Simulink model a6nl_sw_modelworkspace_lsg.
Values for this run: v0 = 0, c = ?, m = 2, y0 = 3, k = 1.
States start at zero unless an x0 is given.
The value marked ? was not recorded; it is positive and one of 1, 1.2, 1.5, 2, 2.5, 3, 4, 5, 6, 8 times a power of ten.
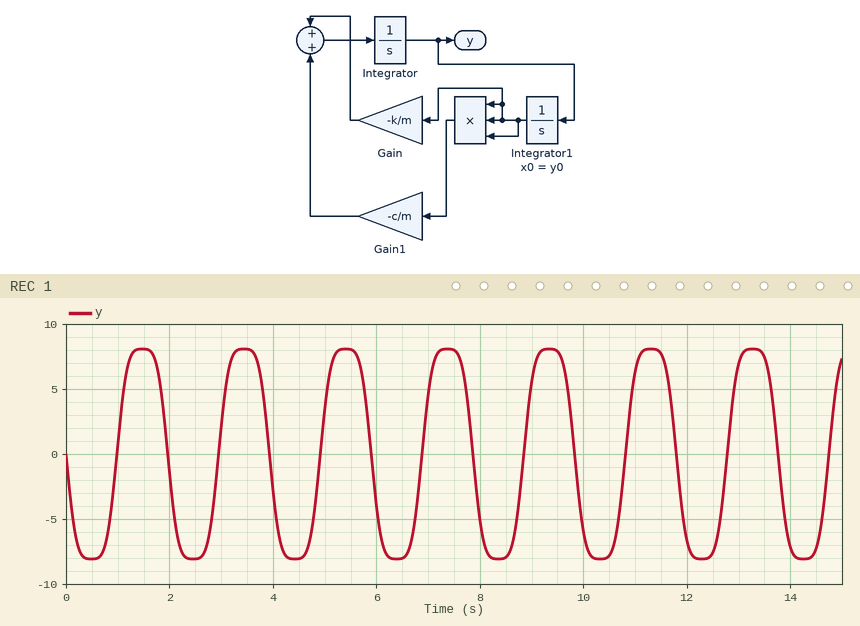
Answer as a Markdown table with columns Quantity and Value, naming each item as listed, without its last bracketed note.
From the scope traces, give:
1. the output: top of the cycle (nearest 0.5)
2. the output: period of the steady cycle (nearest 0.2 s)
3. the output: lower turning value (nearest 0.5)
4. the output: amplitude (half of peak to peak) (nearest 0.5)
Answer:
| Quantity | Value |
|---|---|
| the output: top of the cycle | 8.0 |
| the output: period of the steady cycle | 2.0 s |
| the output: lower turning value | -8.0 |
| the output: amplitude (half of peak to peak) | 8.0 |
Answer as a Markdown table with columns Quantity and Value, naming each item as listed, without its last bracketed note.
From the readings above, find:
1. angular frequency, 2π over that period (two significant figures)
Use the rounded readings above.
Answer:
| Quantity | Value |
|---|---|
| angular frequency, 2π over that period | 3.1 rad/s |
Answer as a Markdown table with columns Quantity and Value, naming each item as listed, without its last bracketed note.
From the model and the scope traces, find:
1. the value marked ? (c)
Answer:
| Quantity | Value |
|---|---|
| the value marked ? | 3 |
